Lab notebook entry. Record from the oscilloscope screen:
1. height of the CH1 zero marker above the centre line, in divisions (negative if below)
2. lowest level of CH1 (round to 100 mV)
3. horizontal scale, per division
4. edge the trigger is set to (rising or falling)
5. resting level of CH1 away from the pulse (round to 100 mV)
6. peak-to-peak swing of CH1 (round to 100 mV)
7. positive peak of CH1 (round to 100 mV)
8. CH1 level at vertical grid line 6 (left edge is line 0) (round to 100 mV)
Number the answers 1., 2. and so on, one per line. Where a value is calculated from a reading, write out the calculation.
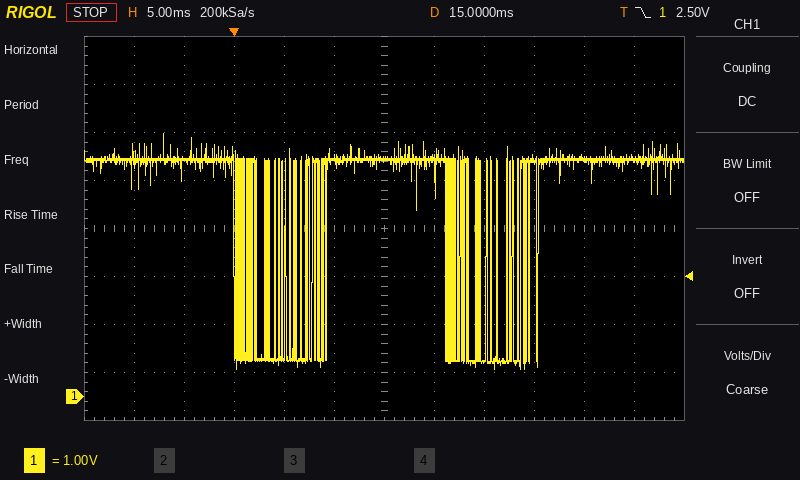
1. -3.5 div
2. 600 mV
3. 5 ms
4. falling
5. 4.9 V
6. 5.5 V − (600 mV) = 4.9 V
7. 5.5 V
8. 4.9 V
